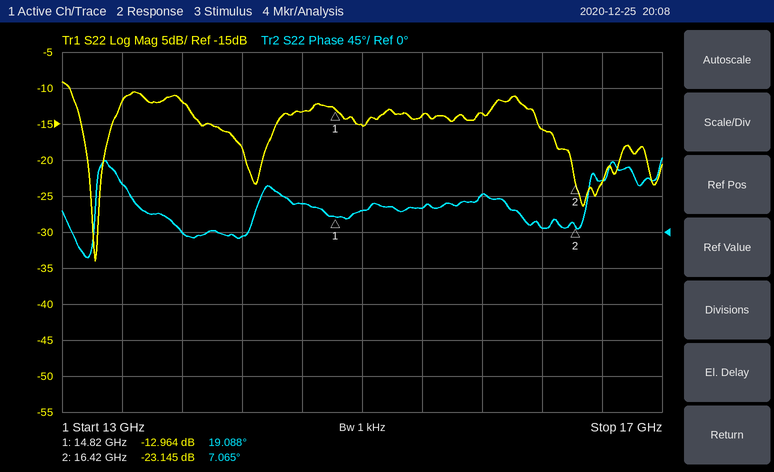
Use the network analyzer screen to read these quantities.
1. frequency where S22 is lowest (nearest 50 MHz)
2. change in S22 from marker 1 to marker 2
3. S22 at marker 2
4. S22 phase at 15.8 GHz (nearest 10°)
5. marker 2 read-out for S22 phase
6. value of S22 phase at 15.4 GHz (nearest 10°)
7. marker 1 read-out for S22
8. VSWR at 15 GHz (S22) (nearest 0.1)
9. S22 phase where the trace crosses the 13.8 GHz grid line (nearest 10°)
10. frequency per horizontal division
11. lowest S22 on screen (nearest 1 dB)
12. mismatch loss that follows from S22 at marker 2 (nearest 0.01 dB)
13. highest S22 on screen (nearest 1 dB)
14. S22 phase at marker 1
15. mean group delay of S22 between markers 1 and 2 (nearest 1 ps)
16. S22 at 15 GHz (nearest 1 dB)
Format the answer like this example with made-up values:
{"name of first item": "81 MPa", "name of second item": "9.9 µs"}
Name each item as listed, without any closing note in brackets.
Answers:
{"frequency where S22 is lowest": "13.20 GHz", "change in S22 from marker 1 to marker 2": "-10.181 dB", "S22 at marker 2": "-23.145 dB", "S22 phase at 15.8 GHz": "50°", "marker 2 read-out for S22 phase": "7.065°", "value of S22 phase at 15.4 GHz": "30°", "marker 1 read-out for S22": "-12.964 dB", "VSWR at 15 GHz (S22)": "1.4", "S22 phase where the trace crosses the 13.8 GHz grid line": "0°", "frequency per horizontal division": "400 MHz", "lowest S22 on screen": "-34 dB", "mismatch loss that follows from S22 at marker 2": "0.02 dB", "highest S22 on screen": "-9 dB", "S22 phase at marker 1": "19.088°", "mean group delay of S22 between markers 1 and 2": "21 ps", "S22 at 15 GHz": "-15 dB"}
